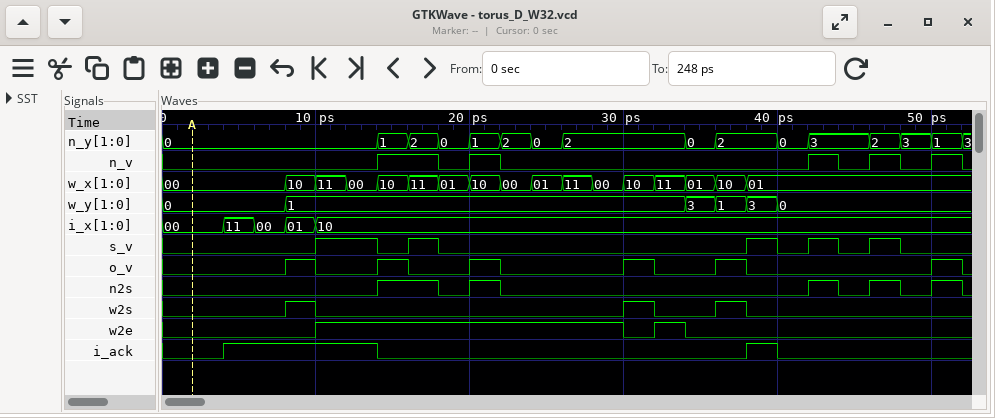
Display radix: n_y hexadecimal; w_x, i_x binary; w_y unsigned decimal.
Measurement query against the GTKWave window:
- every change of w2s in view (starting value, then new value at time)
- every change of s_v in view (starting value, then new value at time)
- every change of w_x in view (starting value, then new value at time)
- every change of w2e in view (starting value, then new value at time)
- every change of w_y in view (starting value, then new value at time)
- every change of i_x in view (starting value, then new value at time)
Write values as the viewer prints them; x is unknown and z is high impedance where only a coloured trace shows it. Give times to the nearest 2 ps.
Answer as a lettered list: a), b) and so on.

a) 0, 1 at 8 ps, 0 at 10 ps, 1 at 30 ps, 0 at 32 ps, 1 at 36 ps, 0 at 38 ps
b) 0, 1 at 10 ps, 0 at 14 ps, 1 at 16 ps, 0 at 18 ps, 1 at 38 ps, 0 at 40 ps, 1 at 42 ps, 0 at 44 ps, 1 at 46 ps, 0 at 48 ps
c) 00, 10 at 8 ps, 11 at 10 ps, 00 at 12 ps, 10 at 14 ps, 11 at 16 ps, 01 at 18 ps, 10 at 20 ps, 00 at 22 ps, 01 at 24 ps, 11 at 26 ps, 00 at 28 ps, 10 at 30 ps, 11 at 32 ps, 01 at 34 ps, 10 at 36 ps, 01 at 38 ps
d) 0, 1 at 10 ps, 0 at 30 ps, 1 at 32 ps, 0 at 34 ps
e) 0, 1 at 8 ps, 3 at 34 ps, 1 at 36 ps, 3 at 38 ps, 0 at 40 ps
f) 00, 11 at 4 ps, 00 at 6 ps, 01 at 8 ps, 10 at 10 ps
